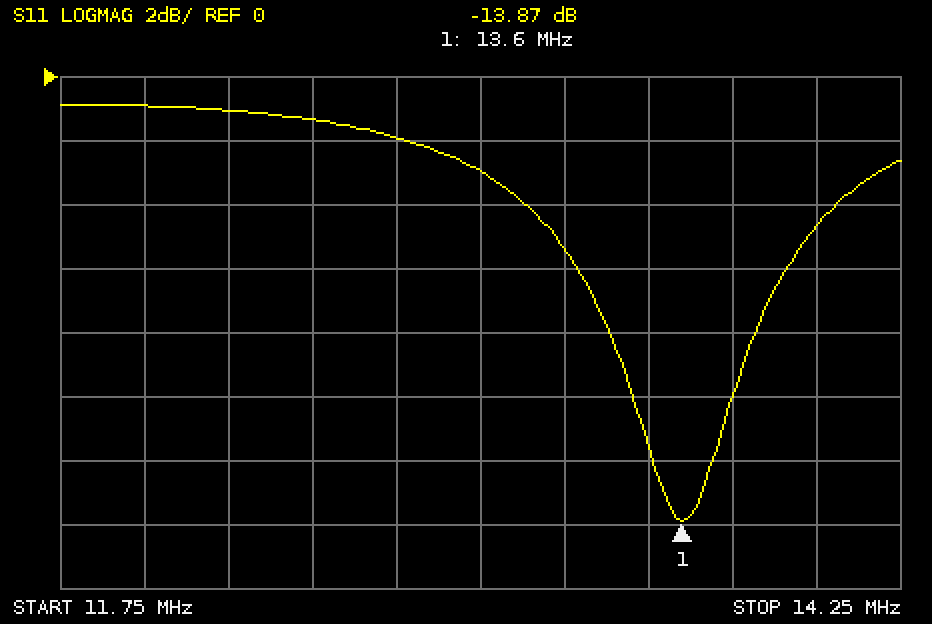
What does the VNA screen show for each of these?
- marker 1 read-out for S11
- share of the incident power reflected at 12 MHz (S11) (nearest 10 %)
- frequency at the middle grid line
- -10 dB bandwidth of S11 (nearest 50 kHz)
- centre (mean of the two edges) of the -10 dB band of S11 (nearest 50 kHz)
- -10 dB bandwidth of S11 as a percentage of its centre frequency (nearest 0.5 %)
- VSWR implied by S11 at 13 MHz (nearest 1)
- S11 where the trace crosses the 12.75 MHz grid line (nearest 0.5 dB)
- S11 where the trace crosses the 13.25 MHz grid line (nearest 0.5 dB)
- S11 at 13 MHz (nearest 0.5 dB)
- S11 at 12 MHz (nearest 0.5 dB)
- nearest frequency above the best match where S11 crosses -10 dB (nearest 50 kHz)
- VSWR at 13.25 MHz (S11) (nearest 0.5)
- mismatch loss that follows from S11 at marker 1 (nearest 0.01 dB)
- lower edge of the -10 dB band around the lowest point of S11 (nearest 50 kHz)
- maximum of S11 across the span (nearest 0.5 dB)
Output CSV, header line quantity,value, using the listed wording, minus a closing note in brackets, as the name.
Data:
quantity,value
marker 1 read-out for S11,-13.87 dB
share of the incident power reflected at 12 MHz (S11),80 %
frequency at the middle grid line,13 MHz
-10 dB bandwidth of S11,300 kHz
centre (mean of the two edges) of the -10 dB band of S11,13.60 MHz
-10 dB bandwidth of S11 as a percentage of its centre frequency,2.0 %
VSWR implied by S11 at 13 MHz,6
S11 where the trace crosses the 12.75 MHz grid line,-2.0 dB
S11 where the trace crosses the 13.25 MHz grid line,-5.5 dB
S11 at 13 MHz,-3.0 dB
S11 at 12 MHz,-1.0 dB
nearest frequency above the best match where S11 crosses -10 dB,13.75 MHz
VSWR at 13.25 MHz (S11),3.5
mismatch loss that follows from S11 at marker 1,0.18 dB
lower edge of the -10 dB band around the lowest point of S11,13.45 MHz
maximum of S11 across the span,-1.0 dB
